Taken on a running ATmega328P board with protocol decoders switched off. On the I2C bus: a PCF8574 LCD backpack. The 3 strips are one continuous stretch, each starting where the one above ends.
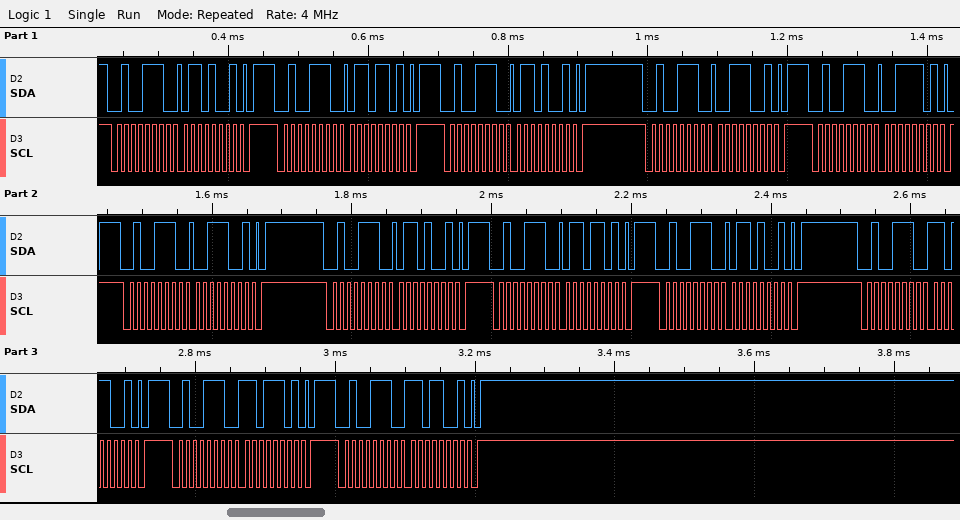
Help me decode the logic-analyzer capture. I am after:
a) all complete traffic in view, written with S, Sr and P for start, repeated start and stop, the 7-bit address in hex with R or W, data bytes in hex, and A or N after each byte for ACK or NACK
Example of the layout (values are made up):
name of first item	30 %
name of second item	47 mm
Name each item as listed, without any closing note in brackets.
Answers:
all complete traffic in view, written with S, Sr and P for start, repeated start and stop, the 7-bit address in hex with R or W, data bytes in hex, and A or N after each byte for ACK or NACK	S 27W A 69 A P S 27W A 6D A P S 27W A 69 A P S 27W A 39 A P S 27W A 3D A P S 27W A 39 A P S 27W A 69 A P S 27W A 6D A P S 27W A 69 A P S 27W A D9 A P S 27W A DD A P S 27W A D9 A P
